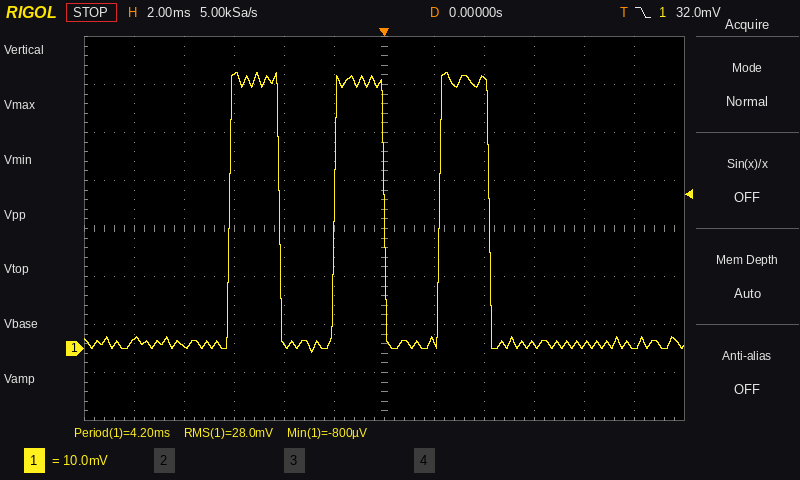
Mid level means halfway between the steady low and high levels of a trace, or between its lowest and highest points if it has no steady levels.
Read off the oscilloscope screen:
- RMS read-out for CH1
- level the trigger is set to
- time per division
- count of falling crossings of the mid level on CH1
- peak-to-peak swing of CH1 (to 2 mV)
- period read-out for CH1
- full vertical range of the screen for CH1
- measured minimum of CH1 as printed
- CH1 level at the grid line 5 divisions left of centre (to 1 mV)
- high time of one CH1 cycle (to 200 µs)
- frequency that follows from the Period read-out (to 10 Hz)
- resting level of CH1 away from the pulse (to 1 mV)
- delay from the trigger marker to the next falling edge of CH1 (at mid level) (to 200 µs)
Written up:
28.0 mV
32.0 mV
2 ms
3
58 mV
4.20 ms
80 mV
-800 µV
2 mV
2.0 ms
240 Hz
1 mV
4.2 ms
